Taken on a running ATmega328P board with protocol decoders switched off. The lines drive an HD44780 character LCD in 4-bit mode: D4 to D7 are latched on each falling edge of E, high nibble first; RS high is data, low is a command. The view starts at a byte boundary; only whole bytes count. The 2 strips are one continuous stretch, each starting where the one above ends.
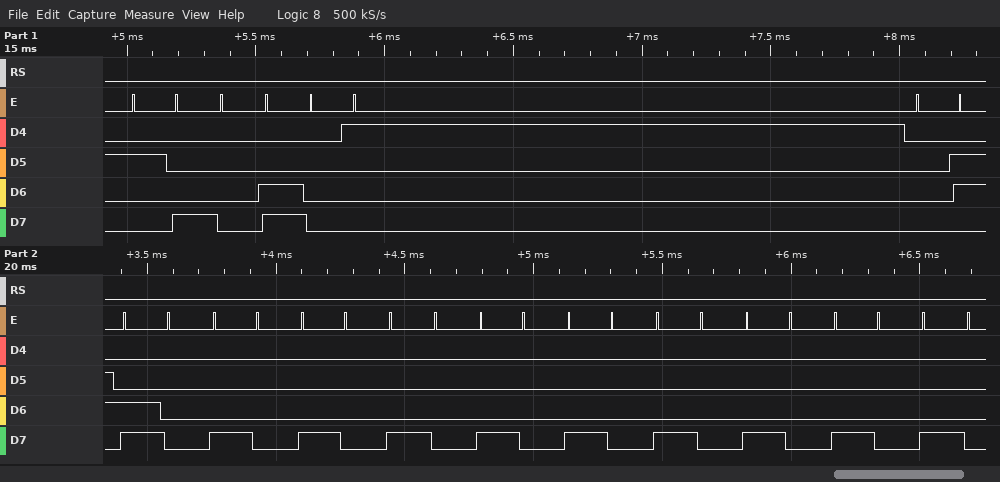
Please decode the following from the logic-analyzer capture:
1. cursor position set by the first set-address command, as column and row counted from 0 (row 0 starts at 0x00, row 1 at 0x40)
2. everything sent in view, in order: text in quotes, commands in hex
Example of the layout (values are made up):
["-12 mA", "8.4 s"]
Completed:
["column 0, row 1", "0x28 0x0C 0x01 0x06 0xC0 0x80 0x80 0x80 0x80 0x80 0x80 0x80 0x80 0x80"]
